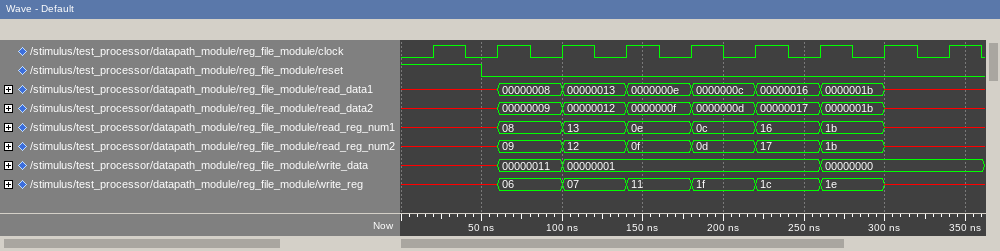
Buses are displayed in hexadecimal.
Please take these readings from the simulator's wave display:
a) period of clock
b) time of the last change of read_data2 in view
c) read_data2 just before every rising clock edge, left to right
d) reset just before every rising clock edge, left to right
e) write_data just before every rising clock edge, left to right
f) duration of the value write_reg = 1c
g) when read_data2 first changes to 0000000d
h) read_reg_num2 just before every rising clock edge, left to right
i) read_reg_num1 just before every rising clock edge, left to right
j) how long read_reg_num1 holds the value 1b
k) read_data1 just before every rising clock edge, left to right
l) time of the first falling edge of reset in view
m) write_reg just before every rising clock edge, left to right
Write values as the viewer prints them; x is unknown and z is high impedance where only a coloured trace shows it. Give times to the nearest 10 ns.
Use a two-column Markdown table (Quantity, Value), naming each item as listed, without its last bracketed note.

| Quantity | Value |
|---|---|
| period of clock | 40 ns |
| time of the last change of read_data2 in view | 300 ns |
| read_data2 just before every rising clock edge, left to right | x, x, 00000009, 00000012, 0000000f, 0000000d, 00000017, 0000001b, x |
| reset just before every rising clock edge, left to right | 1 0 0 0 0 0 0 0 0 |
| write_data just before every rising clock edge, left to right | x, x, 00000011, 00000001, 00000001, 00000001, 00000001, 00000000, 00000000 |
| duration of the value write_reg = 1c | 40 ns |
| when read_data2 first changes to 0000000d | 180 ns |
| read_reg_num2 just before every rising clock edge, left to right | x, x, 09, 12, 0f, 0d, 17, 1b, x |
| read_reg_num1 just before every rising clock edge, left to right | x, x, 08, 13, 0e, 0c, 16, 1b, x |
| how long read_reg_num1 holds the value 1b | 40 ns |
| read_data1 just before every rising clock edge, left to right | x, x, 00000008, 00000013, 0000000e, 0000000c, 00000016, 0000001b, x |
| time of the first falling edge of reset in view | 50 ns |
| write_reg just before every rising clock edge, left to right | x, x, 06, 07, 11, 1f, 1c, 1e, x |
